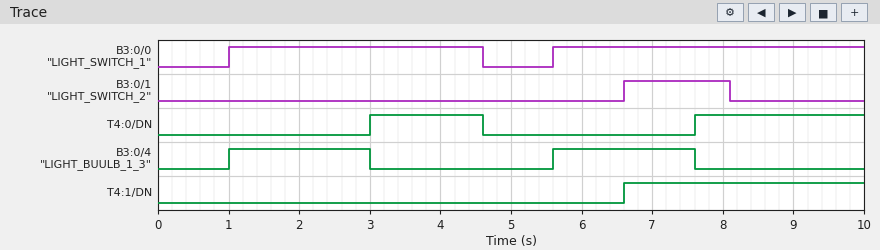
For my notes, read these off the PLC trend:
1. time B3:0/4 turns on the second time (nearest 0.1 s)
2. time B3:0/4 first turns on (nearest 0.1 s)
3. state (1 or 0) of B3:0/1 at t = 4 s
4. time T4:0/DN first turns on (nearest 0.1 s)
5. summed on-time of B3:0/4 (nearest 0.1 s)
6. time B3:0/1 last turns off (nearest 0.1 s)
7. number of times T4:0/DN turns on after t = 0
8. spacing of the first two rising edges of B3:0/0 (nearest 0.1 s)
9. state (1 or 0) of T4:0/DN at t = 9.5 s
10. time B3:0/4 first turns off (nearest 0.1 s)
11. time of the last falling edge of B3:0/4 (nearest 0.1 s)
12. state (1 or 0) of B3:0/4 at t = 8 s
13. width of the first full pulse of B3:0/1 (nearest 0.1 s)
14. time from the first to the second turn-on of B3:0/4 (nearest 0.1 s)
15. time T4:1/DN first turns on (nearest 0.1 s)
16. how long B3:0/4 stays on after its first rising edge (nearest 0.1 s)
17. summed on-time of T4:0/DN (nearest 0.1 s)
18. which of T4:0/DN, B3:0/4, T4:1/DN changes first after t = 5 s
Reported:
5.6 s
1.0 s
0
3.0 s
4.0 s
8.1 s
2
4.6 s
1
3.0 s
7.6 s
0
1.5 s
4.6 s
6.6 s
2.0 s
4.0 s
B3:0/4
